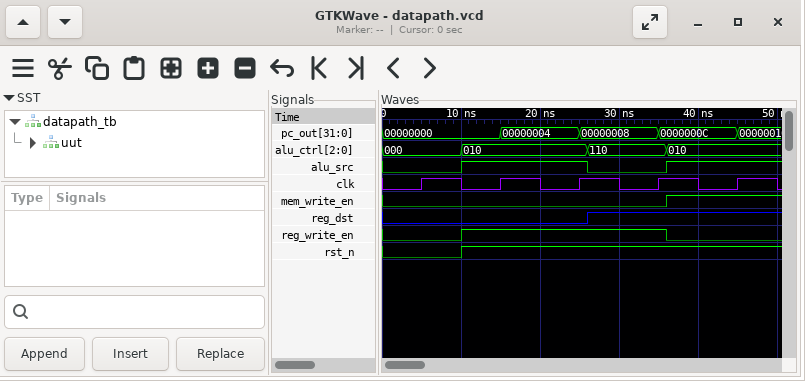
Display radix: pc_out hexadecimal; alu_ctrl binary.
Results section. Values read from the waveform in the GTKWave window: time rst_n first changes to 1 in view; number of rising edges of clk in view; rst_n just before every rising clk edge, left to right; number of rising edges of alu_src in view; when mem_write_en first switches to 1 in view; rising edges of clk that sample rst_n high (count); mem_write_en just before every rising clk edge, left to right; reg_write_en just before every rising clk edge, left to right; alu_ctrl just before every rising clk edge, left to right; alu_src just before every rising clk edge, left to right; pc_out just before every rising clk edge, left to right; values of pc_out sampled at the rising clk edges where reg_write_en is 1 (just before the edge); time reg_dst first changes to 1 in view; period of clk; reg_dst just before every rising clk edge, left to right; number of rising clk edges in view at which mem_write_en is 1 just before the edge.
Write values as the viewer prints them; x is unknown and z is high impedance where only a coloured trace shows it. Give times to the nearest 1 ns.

10 ns
5
0 1 1 1 1
2
36 ns
4
0 0 0 0 1
0 1 1 1 0
000, 010, 010, 110, 010
0 1 1 0 1
00000000, 00000000, 00000004, 00000008, 0000000C
00000000, 00000004, 00000008
26 ns
10 ns
0 0 0 1 1
1
